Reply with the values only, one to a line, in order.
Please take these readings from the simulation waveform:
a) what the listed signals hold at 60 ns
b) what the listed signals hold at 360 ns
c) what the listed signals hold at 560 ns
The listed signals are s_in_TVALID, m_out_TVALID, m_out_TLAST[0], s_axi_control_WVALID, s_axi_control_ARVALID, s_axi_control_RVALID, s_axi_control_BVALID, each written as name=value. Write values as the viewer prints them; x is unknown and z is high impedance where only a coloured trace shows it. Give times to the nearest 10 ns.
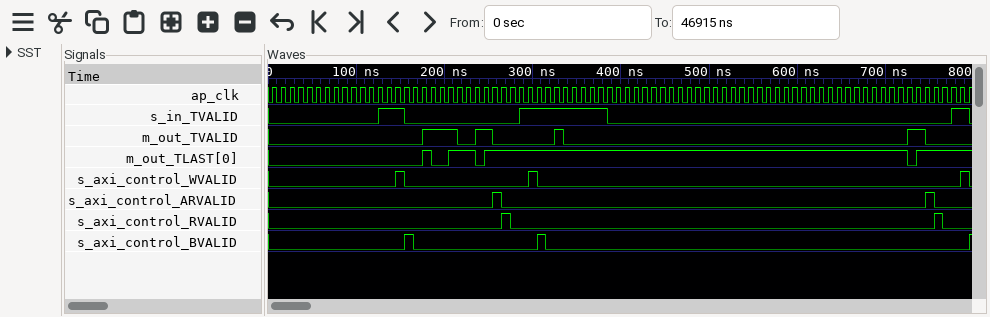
s_in_TVALID=0, m_out_TVALID=0, m_out_TLAST[0]=0, s_axi_control_WVALID=0, s_axi_control_ARVALID=0, s_axi_control_RVALID=0, s_axi_control_BVALID=0
s_in_TVALID=1, m_out_TVALID=0, m_out_TLAST[0]=1, s_axi_control_WVALID=0, s_axi_control_ARVALID=0, s_axi_control_RVALID=0, s_axi_control_BVALID=0
s_in_TVALID=0, m_out_TVALID=0, m_out_TLAST[0]=1, s_axi_control_WVALID=0, s_axi_control_ARVALID=0, s_axi_control_RVALID=0, s_axi_control_BVALID=0
